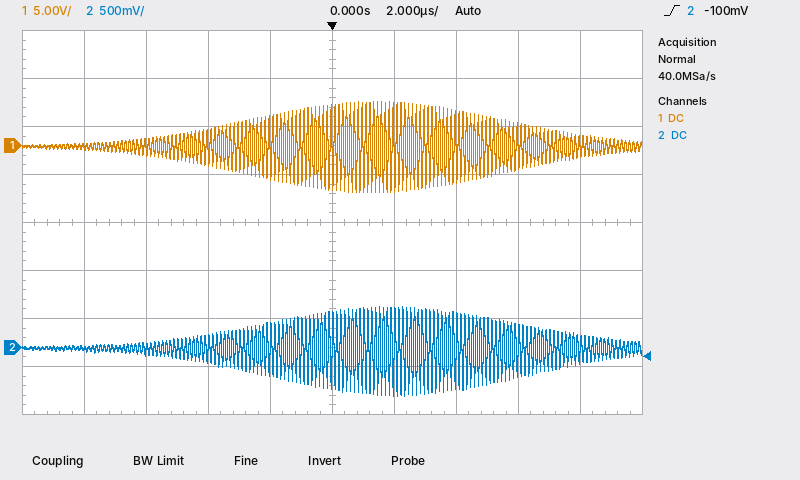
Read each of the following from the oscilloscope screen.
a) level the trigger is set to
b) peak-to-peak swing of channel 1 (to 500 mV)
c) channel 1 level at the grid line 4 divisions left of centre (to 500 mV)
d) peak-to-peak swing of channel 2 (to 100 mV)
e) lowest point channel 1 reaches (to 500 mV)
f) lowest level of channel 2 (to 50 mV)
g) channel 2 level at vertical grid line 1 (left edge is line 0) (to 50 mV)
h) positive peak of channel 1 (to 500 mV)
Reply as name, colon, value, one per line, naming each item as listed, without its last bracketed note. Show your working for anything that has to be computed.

level the trigger is set to: -100 mV
peak-to-peak swing of channel 1: 4.5 V − (-5.0 V) = 9.5 V
channel 1 level at the grid line 4 divisions left of centre: 0.0 V
peak-to-peak swing of channel 2: 900 mV
lowest point channel 1 reaches: -5.0 V
lowest level of channel 2: -500 mV
channel 2 level at vertical grid line 1 (left edge is line 0): 0 mV
positive peak of channel 1: 4.5 V
